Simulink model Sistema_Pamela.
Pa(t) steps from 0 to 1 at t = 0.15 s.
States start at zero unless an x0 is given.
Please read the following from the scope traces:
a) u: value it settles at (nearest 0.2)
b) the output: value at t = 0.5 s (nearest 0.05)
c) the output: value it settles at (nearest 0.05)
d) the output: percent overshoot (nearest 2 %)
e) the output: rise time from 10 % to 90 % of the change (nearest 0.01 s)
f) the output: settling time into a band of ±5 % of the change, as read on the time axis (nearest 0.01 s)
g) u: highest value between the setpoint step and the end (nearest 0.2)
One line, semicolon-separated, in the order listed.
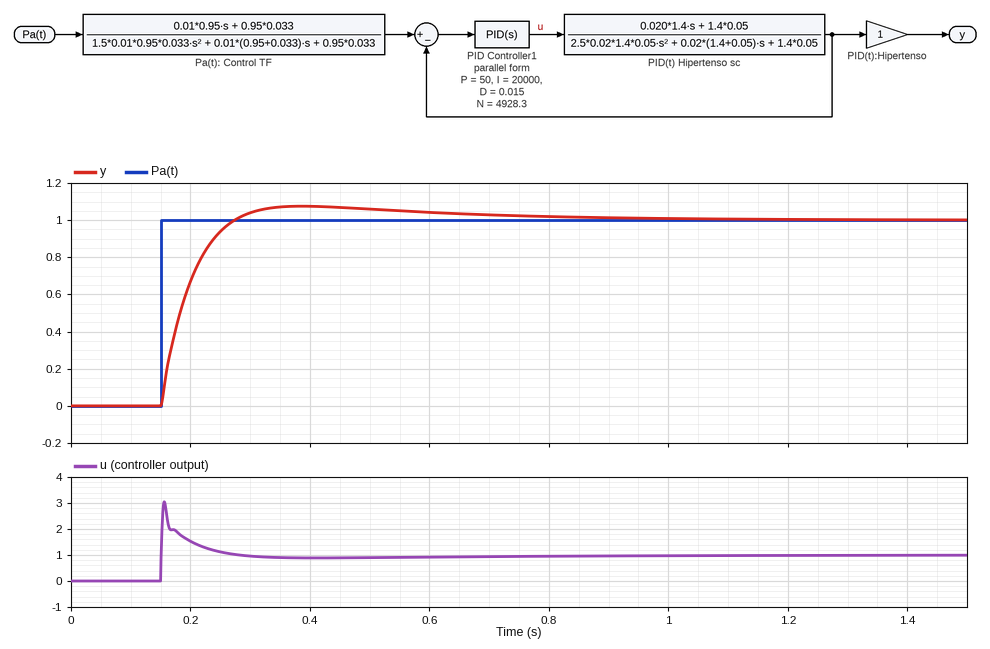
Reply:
1.0; 1.05; 1.00; 8 %; 0.08 s; 0.55 s; 3.0
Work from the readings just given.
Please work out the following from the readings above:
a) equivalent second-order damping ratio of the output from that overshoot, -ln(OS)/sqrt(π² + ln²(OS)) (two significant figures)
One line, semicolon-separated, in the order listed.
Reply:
0.63
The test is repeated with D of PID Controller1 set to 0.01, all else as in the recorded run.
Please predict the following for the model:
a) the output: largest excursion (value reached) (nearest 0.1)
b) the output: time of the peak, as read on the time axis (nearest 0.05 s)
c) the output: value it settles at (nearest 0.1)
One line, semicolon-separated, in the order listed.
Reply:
1.1; 0.40 s; 1.0
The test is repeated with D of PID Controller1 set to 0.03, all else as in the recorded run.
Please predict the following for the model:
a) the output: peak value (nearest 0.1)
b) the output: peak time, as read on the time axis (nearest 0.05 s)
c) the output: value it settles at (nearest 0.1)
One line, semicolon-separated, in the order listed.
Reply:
1.1; 0.40 s; 1.0
